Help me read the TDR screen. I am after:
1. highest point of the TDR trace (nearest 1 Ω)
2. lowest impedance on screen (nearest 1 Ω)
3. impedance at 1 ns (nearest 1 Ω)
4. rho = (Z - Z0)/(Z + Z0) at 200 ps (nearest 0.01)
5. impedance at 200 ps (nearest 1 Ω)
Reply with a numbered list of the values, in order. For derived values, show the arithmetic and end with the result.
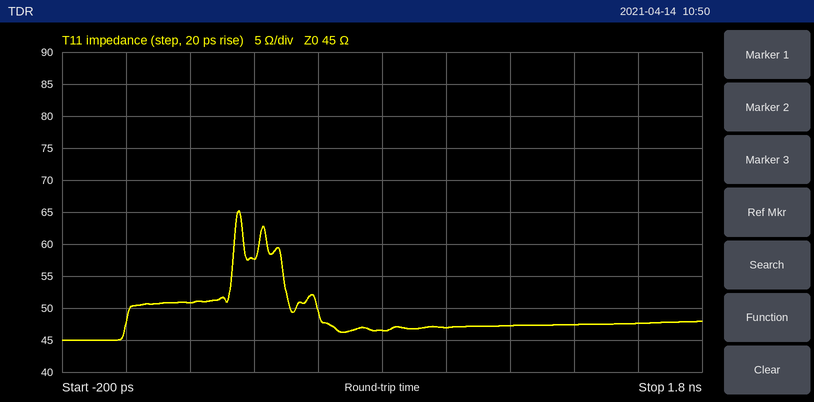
1. 65 Ω
2. 45 Ω
3. 47 Ω
4. (51 − 45)/(51 + 45) ≈ +0.06
5. 51 Ω
